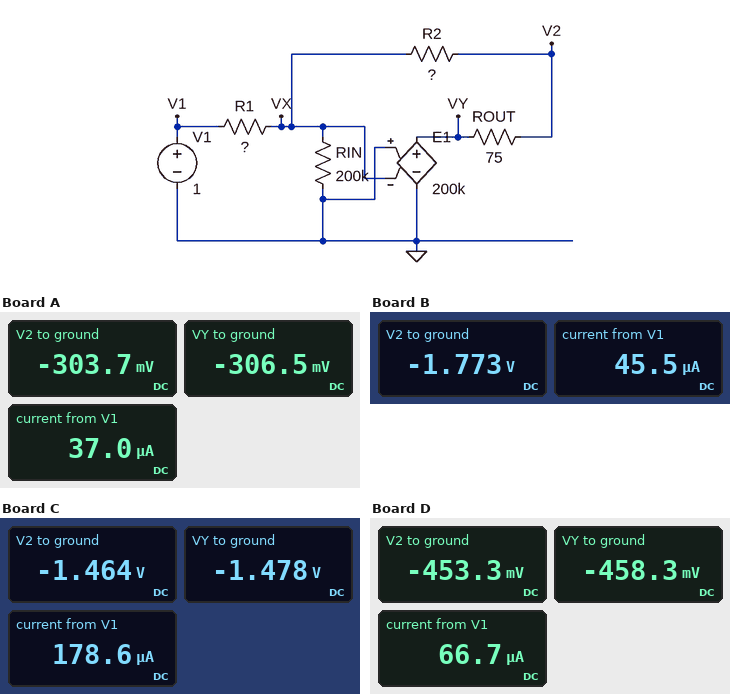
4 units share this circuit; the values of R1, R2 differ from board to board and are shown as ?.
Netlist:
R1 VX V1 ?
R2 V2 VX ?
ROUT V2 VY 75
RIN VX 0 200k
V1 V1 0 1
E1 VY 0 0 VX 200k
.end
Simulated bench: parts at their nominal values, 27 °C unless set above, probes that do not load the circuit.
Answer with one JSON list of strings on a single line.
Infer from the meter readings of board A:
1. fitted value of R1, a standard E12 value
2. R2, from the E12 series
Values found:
["27 kΩ", "8.2 kΩ"]
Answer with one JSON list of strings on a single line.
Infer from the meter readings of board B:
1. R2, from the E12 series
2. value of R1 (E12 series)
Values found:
["39 kΩ", "22 kΩ"]
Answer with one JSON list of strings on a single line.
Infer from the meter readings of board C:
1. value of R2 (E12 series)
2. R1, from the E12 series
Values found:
["8.2 kΩ", "5.6 kΩ"]
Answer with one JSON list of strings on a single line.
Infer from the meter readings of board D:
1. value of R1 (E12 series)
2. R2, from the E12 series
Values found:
["15 kΩ", "6.8 kΩ"]
